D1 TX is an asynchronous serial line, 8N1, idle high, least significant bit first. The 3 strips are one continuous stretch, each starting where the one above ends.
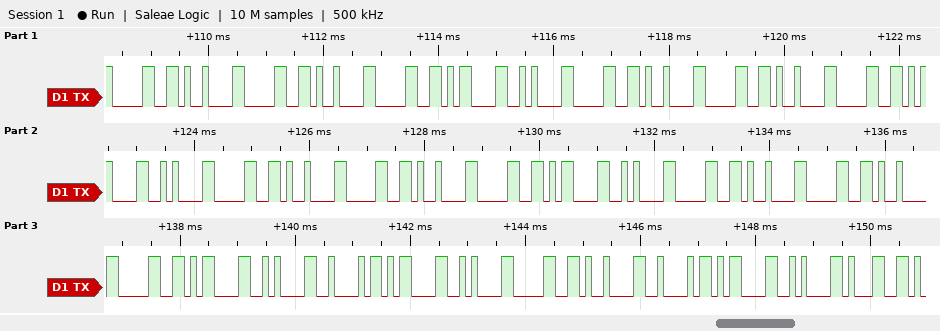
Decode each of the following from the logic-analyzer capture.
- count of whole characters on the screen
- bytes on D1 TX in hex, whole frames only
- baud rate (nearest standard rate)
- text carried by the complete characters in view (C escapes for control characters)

37
30 09 30 09 30 0D 0A 30 09 30 09 30 0D 0A 30 09 30 09 30 0D 0A 30 09 30 09 30 0D 0A 42 0D 0A 30 09 42 0D 0A 31
9600 baud
"0\t0\t0\r\n0\t0\t0\r\n0\t0\t0\r\n0\t0\t0\r\nB\r\n0\tB\r\n1"
